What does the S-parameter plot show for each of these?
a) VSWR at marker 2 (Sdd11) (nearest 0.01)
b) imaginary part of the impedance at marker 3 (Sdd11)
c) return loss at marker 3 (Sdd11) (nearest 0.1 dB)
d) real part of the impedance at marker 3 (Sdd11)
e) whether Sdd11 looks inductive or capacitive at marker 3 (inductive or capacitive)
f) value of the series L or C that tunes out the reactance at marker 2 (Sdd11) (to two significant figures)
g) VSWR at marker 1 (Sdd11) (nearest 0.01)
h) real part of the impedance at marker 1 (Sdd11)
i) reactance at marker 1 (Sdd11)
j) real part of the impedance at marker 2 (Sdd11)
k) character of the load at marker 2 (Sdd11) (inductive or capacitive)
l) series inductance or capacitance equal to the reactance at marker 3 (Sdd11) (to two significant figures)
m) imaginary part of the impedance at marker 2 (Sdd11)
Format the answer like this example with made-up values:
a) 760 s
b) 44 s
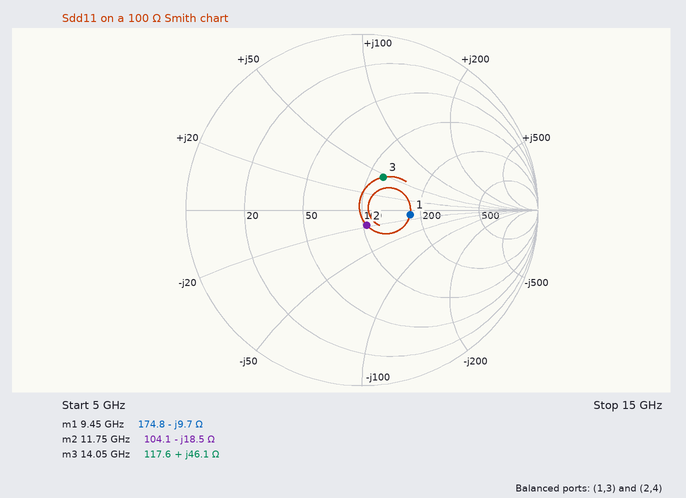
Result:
a) 1.20
b) +46.1 Ω
c) 13.1 dB
d) 117.6 Ω
e) inductive
f) 250 pH
g) 1.76
h) 174.8 Ω
i) -9.7 Ω
j) 104.1 Ω
k) capacitive
l) 520 pH
m) -18.5 Ω
